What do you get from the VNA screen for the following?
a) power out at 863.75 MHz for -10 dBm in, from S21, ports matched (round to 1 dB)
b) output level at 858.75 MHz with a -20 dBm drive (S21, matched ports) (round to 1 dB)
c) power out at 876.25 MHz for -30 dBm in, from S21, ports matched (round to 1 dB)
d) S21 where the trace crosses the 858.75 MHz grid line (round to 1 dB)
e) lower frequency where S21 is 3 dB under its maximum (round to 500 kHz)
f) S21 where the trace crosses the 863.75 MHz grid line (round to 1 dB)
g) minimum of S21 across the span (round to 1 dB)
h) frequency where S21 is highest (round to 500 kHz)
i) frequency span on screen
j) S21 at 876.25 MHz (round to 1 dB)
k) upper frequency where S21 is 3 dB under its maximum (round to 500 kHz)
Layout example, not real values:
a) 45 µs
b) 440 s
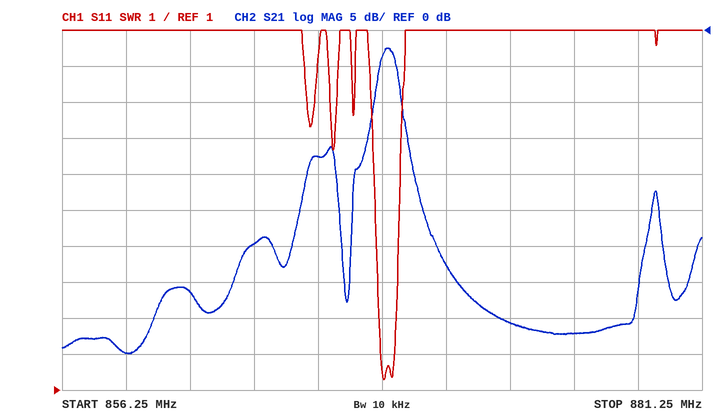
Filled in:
a) -40 dBm
b) -65 dBm
c) -72 dBm
d) -45 dB
e) 868.5 MHz
f) -30 dB
g) -45 dB
h) 869.0 MHz
i) 25 MHz
j) -42 dB
k) 869.5 MHz
